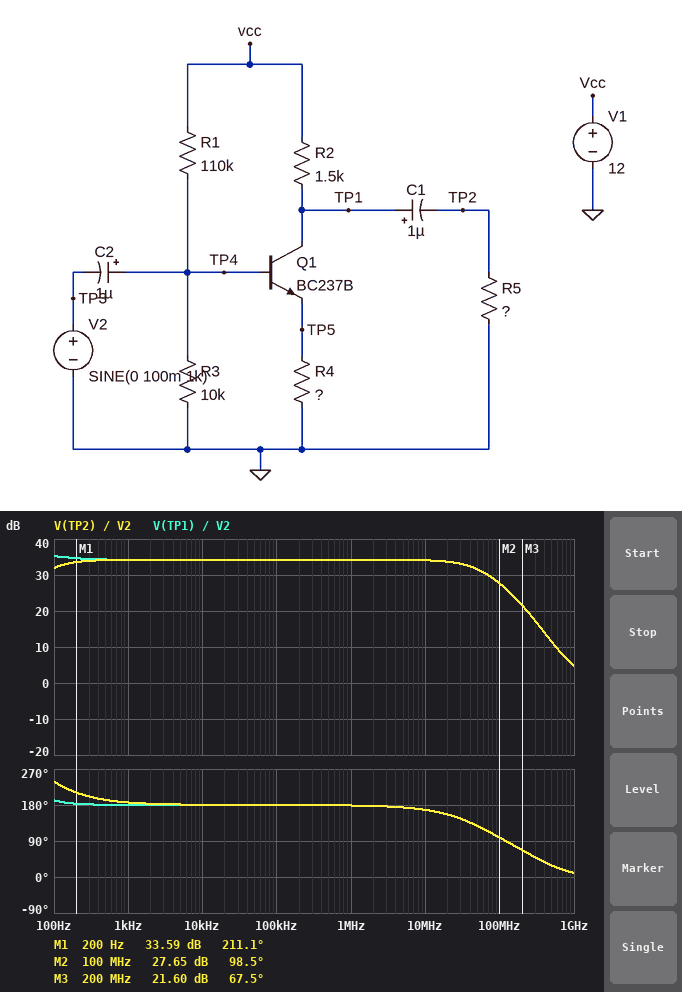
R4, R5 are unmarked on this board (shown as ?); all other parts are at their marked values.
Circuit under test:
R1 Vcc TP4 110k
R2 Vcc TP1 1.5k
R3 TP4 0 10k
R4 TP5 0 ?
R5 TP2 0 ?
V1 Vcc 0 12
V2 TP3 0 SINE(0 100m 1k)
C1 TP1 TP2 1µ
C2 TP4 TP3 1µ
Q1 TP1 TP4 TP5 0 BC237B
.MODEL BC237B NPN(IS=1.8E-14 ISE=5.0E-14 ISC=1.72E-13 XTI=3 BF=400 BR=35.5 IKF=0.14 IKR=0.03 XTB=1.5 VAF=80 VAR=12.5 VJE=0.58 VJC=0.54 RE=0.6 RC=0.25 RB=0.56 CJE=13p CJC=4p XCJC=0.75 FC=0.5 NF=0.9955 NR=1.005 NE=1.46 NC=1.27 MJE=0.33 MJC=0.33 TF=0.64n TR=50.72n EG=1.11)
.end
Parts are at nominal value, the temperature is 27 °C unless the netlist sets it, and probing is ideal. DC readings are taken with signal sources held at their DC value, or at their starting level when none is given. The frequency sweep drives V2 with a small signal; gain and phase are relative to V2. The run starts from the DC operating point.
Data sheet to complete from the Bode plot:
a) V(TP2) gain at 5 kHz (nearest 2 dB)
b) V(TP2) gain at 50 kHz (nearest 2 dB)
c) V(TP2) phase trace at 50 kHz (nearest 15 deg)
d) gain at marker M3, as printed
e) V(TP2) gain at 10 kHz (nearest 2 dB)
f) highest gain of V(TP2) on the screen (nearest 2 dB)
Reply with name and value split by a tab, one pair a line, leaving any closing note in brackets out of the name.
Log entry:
V(TP2) gain at 5 kHz	34 dB
V(TP2) gain at 50 kHz	34 dB
V(TP2) phase trace at 50 kHz	180 deg
gain at marker M3, as printed	21.60 dB
V(TP2) gain at 10 kHz	34 dB
highest gain of V(TP2) on the screen	34 dB
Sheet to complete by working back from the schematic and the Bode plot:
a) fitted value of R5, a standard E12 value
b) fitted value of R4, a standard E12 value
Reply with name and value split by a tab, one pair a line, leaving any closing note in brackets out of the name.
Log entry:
fitted value of R5, a standard E12 value	1.5 kΩ
fitted value of R4, a standard E12 value	10 Ω
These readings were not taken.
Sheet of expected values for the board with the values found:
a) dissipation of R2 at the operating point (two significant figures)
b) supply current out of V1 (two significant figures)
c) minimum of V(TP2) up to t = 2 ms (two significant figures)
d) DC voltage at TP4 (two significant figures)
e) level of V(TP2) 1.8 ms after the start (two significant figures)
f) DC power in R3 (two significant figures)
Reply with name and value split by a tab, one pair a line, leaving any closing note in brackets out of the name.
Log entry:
dissipation of R2 at the operating point	82 mW
supply current out of V1	7.5 mA
minimum of V(TP2) up to t = 2 ms	-2.2 V
DC voltage at TP4	770 mV
level of V(TP2) 1.8 ms after the start	4.2 V
DC power in R3	59 µW
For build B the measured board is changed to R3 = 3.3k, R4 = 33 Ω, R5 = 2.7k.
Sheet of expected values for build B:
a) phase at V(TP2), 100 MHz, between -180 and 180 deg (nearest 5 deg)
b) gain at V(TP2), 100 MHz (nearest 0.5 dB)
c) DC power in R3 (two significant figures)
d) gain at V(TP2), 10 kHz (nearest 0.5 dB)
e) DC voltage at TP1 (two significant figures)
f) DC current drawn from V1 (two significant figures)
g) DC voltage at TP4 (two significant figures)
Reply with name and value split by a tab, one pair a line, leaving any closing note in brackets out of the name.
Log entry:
phase at V(TP2), 100 MHz, between -180 and 180 deg	50 deg
gain at V(TP2), 100 MHz	-3.5 dB
DC power in R3	37 µW
gain at V(TP2), 10 kHz	-64.5 dB
DC voltage at TP1	12 V
DC current drawn from V1	110 µA
DC voltage at TP4	350 mV
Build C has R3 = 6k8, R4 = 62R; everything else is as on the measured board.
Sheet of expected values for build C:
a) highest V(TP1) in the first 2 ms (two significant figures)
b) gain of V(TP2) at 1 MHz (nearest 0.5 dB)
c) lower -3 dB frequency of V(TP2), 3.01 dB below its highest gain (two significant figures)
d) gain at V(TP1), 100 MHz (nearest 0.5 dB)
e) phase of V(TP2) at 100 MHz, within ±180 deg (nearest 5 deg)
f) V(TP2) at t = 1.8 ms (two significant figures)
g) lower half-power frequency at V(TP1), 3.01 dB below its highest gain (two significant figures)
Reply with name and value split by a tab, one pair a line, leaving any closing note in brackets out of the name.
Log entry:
highest V(TP1) in the first 2 ms	11 V
gain of V(TP2) at 1 MHz	18.0 dB
lower -3 dB frequency of V(TP2), 3.01 dB below its highest gain	66 Hz
gain at V(TP1), 100 MHz	15.5 dB
phase of V(TP2) at 100 MHz, within ±180 deg	110 deg
V(TP2) at t = 1.8 ms	570 mV
lower half-power frequency at V(TP1), 3.01 dB below its highest gain	18 Hz
